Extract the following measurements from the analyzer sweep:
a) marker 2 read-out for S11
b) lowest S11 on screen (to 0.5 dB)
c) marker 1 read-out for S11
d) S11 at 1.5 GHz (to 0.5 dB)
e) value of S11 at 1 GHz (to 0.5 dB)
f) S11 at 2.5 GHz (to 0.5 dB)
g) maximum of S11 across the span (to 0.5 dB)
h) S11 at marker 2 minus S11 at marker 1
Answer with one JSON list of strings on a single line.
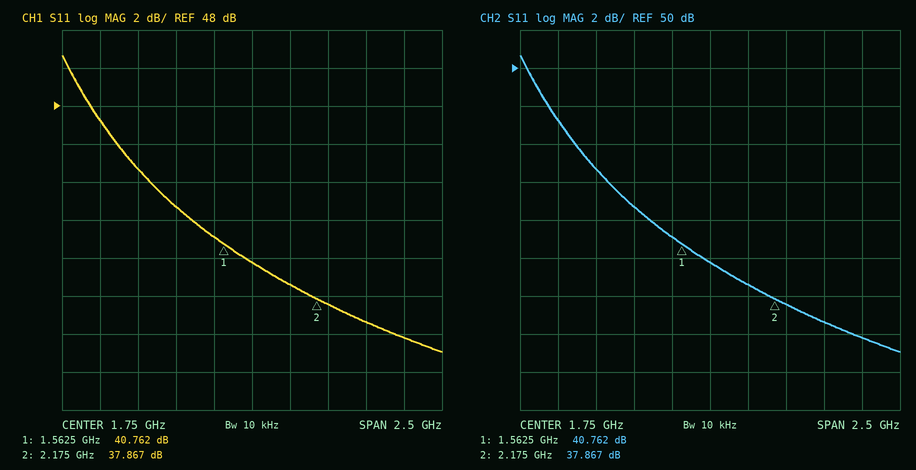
["37.867 dB", "35.0 dB", "40.762 dB", "41.0 dB", "44.5 dB", "36.5 dB", "50.5 dB", "-2.895 dB"]
